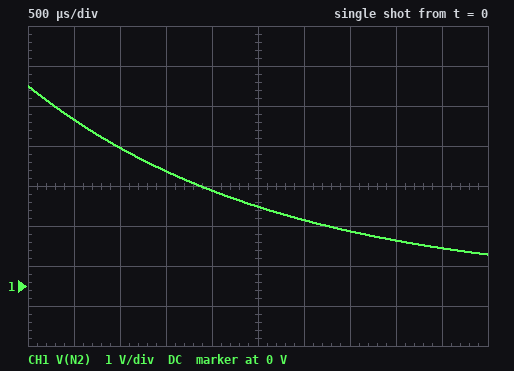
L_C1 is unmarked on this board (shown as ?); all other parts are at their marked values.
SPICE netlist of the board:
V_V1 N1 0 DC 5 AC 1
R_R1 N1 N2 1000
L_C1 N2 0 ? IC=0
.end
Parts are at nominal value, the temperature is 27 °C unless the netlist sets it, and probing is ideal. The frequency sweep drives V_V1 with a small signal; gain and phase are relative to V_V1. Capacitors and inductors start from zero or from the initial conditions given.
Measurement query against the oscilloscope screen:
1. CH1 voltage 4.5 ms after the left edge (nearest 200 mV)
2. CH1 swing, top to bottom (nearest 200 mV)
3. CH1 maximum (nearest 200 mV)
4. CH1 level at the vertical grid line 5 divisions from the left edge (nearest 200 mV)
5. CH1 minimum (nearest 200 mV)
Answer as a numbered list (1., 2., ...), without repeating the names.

1. 1.0 V
2. 4.2 V
3. 5.0 V
4. 2.0 V
5. 800 mV
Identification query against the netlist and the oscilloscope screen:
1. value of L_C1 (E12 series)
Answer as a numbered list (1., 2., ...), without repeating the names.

1. 2.7 H
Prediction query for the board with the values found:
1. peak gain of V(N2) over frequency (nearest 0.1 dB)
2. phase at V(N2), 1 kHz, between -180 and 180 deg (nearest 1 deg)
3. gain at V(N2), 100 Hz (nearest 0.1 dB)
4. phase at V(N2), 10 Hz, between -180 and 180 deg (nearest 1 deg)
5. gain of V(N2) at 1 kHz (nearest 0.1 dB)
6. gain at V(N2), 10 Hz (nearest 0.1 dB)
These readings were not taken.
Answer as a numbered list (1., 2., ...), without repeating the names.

1. 0 dB
2. 3 deg
3. -1.3 dB
4. 80 deg
5. 0 dB
6. -15.5 dB
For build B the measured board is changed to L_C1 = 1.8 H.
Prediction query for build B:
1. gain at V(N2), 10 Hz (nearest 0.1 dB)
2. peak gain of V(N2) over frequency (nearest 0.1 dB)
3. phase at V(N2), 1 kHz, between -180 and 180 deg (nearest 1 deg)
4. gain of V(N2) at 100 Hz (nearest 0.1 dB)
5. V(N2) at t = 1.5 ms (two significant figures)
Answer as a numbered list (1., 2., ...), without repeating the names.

1. -19.0 dB
2. 0 dB
3. 5 deg
4. -2.5 dB
5. 2.2 V
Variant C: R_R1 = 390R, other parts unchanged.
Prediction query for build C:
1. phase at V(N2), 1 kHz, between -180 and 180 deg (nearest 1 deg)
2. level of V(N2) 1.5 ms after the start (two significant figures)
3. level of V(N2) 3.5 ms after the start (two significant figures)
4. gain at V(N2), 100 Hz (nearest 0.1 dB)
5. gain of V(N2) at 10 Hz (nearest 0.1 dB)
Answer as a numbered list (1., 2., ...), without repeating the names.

1. 1 deg
2. 4.0 V
3. 3.0 V
4. -0.2 dB
5. -8.0 dB
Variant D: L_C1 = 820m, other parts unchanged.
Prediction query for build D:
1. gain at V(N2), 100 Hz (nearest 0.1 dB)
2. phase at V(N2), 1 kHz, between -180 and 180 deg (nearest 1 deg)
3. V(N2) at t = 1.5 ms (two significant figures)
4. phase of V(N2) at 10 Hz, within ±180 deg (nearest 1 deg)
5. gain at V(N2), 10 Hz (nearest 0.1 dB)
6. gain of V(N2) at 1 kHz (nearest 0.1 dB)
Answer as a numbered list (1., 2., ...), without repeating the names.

1. -6.8 dB
2. 11 deg
3. 800 mV
4. 87 deg
5. -25.8 dB
6. -0.2 dB
